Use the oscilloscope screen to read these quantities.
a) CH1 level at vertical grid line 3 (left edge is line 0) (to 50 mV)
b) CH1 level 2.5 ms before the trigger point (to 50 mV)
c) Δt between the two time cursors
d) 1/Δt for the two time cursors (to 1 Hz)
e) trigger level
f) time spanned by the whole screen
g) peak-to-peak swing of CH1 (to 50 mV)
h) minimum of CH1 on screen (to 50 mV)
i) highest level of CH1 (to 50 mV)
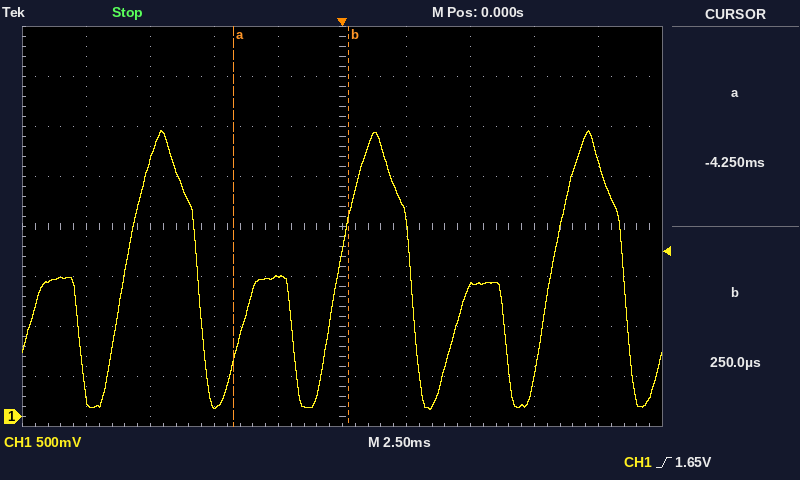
100 mV
1.40 V
4.50 ms
222 Hz
1.65 V
25 ms
2.80 V
50 mV
2.85 V
